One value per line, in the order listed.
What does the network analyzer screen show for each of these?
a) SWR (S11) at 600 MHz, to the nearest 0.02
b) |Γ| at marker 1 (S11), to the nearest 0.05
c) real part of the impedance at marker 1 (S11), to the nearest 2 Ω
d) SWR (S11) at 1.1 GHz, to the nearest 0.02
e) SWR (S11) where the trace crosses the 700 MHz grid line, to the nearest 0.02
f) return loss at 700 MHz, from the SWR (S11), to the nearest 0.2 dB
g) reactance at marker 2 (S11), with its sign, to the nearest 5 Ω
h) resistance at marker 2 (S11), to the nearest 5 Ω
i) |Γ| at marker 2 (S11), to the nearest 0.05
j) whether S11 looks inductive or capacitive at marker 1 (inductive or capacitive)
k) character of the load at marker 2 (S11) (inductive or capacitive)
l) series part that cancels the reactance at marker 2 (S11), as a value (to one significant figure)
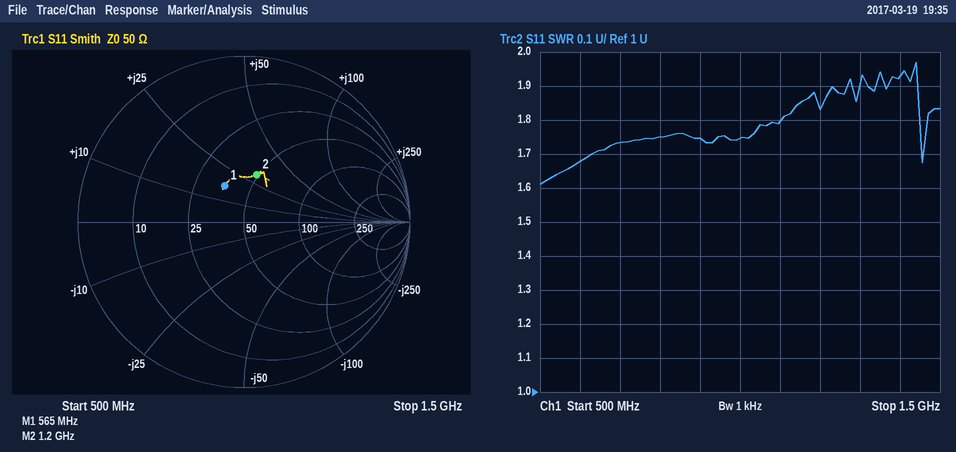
1.68
0.25
36 Ω
1.80
1.74
11.4 dB
+30 Ω
50 Ω
0.30
inductive
inductive
4 pF
